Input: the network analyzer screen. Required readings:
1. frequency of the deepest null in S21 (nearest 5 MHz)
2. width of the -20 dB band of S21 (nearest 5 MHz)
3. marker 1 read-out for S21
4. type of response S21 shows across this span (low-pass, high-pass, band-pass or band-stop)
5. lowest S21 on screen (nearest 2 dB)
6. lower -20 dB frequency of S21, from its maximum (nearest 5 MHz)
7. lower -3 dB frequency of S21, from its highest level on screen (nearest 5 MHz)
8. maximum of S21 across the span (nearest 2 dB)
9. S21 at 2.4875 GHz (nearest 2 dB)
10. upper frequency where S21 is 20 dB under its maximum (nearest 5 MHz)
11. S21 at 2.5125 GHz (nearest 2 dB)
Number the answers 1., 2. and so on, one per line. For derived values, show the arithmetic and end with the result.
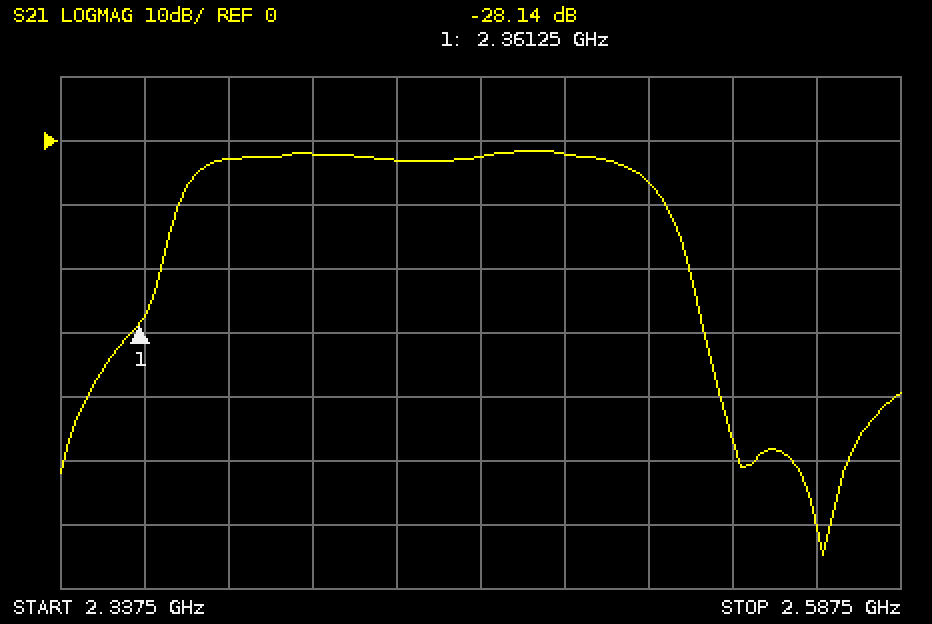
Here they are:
1. 2.565 GHz
2. 2.525 GHz − 2.365 GHz = 160 MHz
3. -28.14 dB
4. band-pass
5. -64 dB
6. 2.365 GHz
7. 2.380 GHz
8. -2 dB
9. -2 dB
10. 2.525 GHz
11. -6 dB
